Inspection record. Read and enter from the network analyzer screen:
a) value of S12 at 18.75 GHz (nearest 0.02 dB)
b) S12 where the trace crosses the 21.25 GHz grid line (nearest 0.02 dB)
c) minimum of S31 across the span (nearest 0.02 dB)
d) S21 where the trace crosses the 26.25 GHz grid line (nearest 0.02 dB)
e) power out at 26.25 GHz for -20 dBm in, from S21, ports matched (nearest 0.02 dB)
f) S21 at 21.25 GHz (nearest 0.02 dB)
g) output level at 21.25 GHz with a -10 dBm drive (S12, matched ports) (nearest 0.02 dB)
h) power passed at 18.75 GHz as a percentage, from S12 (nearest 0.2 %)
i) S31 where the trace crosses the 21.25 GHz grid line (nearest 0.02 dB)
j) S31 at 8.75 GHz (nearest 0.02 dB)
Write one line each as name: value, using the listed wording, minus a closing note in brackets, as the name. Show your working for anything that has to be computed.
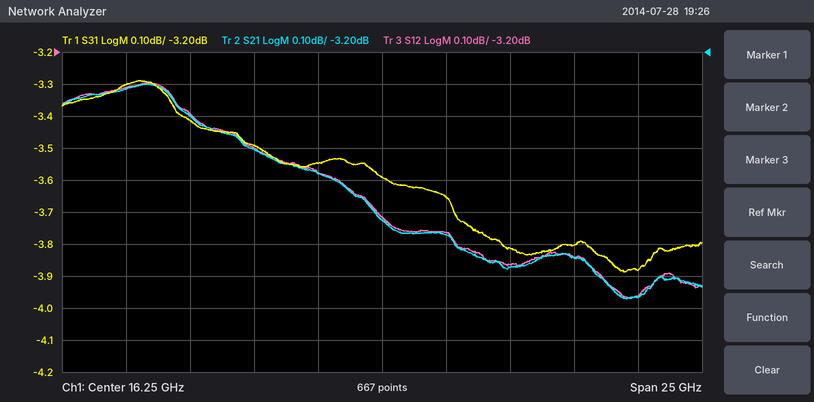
value of S12 at 18.75 GHz: -3.76 dB
S12 where the trace crosses the 21.25 GHz grid line: -3.86 dB
minimum of S31 across the span: -3.88 dB
S21 where the trace crosses the 26.25 GHz grid line: -3.96 dB
power out at 26.25 GHz for -20 dBm in, from S21, ports matched: -20 dBm + (-3.96 dB) = -23.96 dBm
S21 at 21.25 GHz: -3.88 dB
output level at 21.25 GHz with a -10 dBm drive (S12, matched ports): -10 dBm + (-3.86 dB) = -13.86 dBm
power passed at 18.75 GHz as a percentage, from S12: 10^(-3.76/10) ≈ 42.1 %, so 42.0 % to the nearest 0.2 %
S31 where the trace crosses the 21.25 GHz grid line: -3.82 dB
S31 at 8.75 GHz: -3.42 dB
